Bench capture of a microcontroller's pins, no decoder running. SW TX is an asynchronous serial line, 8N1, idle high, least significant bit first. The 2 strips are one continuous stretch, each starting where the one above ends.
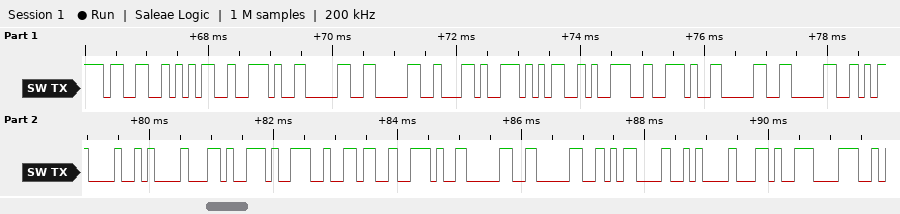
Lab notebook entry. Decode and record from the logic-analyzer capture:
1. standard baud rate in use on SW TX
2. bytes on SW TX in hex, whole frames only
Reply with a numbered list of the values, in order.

1. 9600 baud
2. 0x33 0x35 0x2E 0x30 0x30 0x2C 0x35 0x39 0x2E 0x30 0x30 0x0D 0x0A 0x2C 0x39 0x36 0x2E 0x30 0x30 0x0D 0x0A 0x2C 0x38
